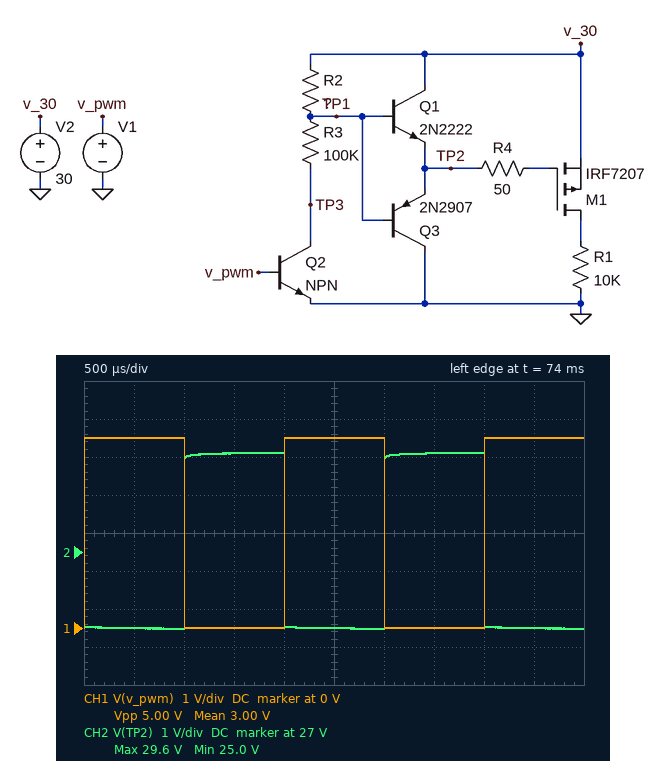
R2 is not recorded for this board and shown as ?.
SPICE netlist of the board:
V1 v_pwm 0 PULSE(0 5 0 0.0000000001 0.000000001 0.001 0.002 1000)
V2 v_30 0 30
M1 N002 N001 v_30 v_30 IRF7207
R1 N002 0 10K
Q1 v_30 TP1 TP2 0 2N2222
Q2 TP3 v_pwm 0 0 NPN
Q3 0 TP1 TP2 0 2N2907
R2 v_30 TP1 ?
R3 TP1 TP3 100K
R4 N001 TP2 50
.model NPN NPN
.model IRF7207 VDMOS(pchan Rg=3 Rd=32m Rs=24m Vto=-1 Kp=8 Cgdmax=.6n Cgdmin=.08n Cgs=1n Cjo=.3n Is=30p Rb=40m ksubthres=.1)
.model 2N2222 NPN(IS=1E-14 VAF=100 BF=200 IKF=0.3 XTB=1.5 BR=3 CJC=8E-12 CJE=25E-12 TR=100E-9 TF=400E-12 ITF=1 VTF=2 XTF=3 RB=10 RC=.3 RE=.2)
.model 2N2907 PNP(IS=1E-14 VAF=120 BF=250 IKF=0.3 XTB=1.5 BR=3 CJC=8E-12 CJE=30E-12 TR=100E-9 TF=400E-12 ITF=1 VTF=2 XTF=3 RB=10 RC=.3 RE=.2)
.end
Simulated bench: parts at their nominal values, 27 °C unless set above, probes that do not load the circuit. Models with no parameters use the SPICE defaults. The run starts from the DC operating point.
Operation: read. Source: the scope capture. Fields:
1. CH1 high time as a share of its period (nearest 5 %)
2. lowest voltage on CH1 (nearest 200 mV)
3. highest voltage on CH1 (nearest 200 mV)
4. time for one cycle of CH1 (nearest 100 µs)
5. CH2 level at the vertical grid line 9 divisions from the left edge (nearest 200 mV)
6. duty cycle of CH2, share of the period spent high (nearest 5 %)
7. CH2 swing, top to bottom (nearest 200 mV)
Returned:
50 %
0 V
5.0 V
2.0 ms
25.0 V
50 %
4.6 V
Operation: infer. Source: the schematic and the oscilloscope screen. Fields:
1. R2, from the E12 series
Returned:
22 kΩ
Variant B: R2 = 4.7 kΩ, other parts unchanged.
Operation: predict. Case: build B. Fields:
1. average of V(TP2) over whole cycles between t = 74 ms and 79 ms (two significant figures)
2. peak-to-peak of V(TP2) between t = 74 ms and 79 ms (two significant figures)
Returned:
29 V
490 mV
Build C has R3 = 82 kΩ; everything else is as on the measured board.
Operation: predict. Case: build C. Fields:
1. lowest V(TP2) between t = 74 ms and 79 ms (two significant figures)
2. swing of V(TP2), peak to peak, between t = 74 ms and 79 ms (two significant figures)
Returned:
24 V
5.6 V
